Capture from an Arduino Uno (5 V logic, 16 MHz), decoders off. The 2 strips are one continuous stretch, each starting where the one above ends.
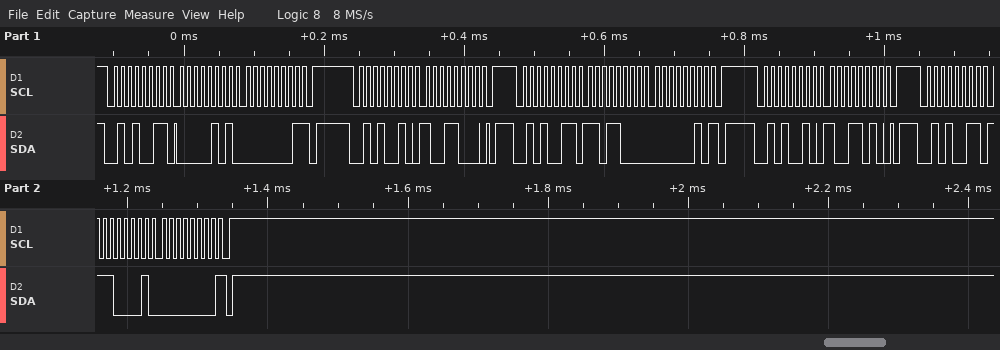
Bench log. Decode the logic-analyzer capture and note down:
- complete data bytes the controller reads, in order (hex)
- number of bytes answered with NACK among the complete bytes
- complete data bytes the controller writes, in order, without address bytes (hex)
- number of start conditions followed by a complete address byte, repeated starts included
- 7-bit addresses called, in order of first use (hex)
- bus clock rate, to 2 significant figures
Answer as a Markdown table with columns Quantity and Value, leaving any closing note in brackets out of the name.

| Quantity | Value |
|---|---|
| complete data bytes the controller reads, in order | 05 01 D8 02 E1 00 |
| number of bytes answered with NACK among the complete bytes | 3 |
| complete data bytes the controller writes, in order, without address bytes | 98 9A |
| number of start conditions followed by a complete address byte, repeated starts included | 5 |
| 7-bit addresses called, in order of first use | 0x29 |
| bus clock rate, to 2 significant figures | 100 kHz |
